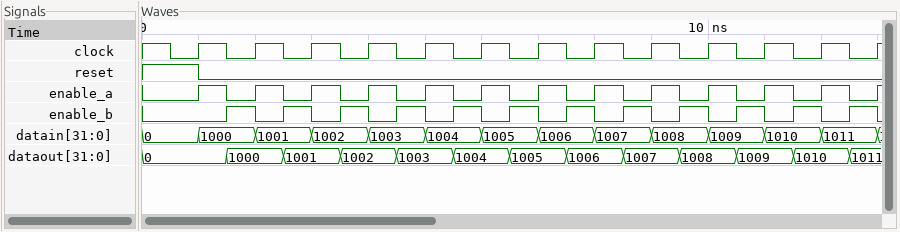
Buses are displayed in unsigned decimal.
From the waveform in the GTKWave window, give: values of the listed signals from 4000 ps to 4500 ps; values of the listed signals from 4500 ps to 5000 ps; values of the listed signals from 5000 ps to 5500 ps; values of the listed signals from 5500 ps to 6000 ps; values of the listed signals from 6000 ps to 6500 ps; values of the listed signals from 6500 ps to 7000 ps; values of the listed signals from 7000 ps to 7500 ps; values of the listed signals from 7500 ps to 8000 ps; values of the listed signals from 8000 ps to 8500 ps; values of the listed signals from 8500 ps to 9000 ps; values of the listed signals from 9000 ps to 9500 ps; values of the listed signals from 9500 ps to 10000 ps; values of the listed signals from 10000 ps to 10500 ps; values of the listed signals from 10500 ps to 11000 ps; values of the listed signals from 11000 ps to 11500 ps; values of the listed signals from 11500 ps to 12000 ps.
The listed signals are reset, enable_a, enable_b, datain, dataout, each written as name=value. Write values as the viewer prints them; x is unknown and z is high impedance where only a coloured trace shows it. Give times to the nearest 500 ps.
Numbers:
reset=0, enable_a=1, enable_b=0, datain=1003, dataout=1002
reset=0, enable_a=0, enable_b=1, datain=1003, dataout=1003
reset=0, enable_a=1, enable_b=0, datain=1004, dataout=1003
reset=0, enable_a=0, enable_b=1, datain=1004, dataout=1004
reset=0, enable_a=1, enable_b=0, datain=1005, dataout=1004
reset=0, enable_a=0, enable_b=1, datain=1005, dataout=1005
reset=0, enable_a=1, enable_b=0, datain=1006, dataout=1005
reset=0, enable_a=0, enable_b=1, datain=1006, dataout=1006
reset=0, enable_a=1, enable_b=0, datain=1007, dataout=1006
reset=0, enable_a=0, enable_b=1, datain=1007, dataout=1007
reset=0, enable_a=1, enable_b=0, datain=1008, dataout=1007
reset=0, enable_a=0, enable_b=1, datain=1008, dataout=1008
reset=0, enable_a=1, enable_b=0, datain=1009, dataout=1008
reset=0, enable_a=0, enable_b=1, datain=1009, dataout=1009
reset=0, enable_a=1, enable_b=0, datain=1010, dataout=1009
reset=0, enable_a=0, enable_b=1, datain=1010, dataout=1010
